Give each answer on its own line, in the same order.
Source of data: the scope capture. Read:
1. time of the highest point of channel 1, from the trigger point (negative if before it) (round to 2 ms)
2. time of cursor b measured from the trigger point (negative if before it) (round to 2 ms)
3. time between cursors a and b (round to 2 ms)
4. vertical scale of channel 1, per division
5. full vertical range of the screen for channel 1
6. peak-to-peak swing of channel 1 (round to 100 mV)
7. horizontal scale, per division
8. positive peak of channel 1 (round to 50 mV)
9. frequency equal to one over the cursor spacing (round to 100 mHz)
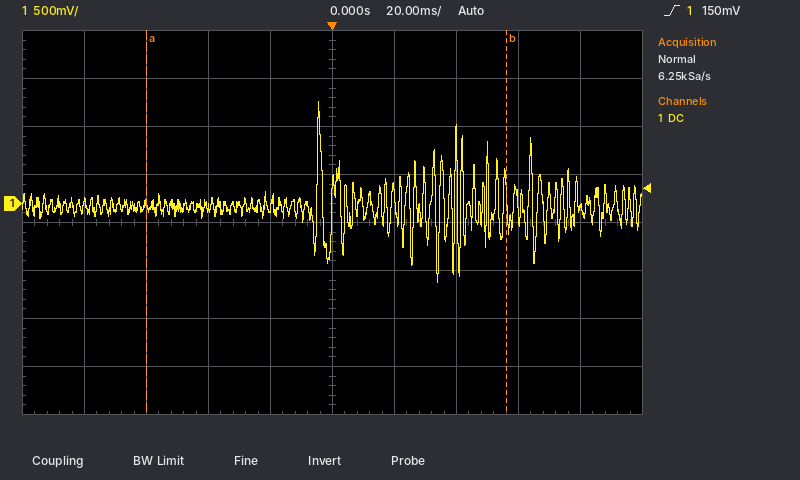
-4 ms
+56 ms
116 ms
500 mV
4 V
1.90 V
20 ms
1.05 V
8.6 Hz
